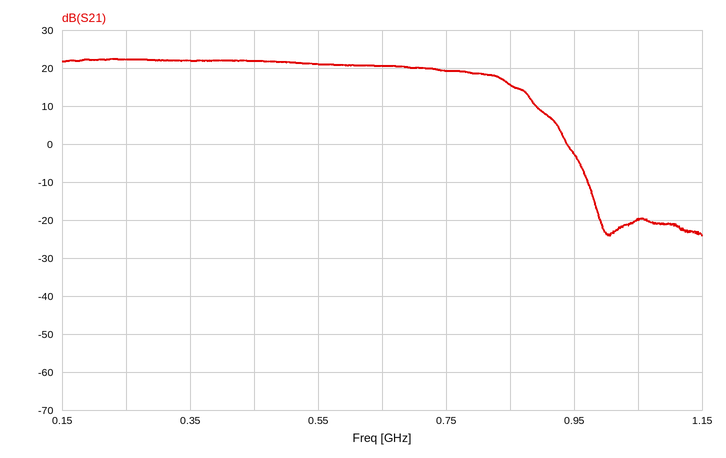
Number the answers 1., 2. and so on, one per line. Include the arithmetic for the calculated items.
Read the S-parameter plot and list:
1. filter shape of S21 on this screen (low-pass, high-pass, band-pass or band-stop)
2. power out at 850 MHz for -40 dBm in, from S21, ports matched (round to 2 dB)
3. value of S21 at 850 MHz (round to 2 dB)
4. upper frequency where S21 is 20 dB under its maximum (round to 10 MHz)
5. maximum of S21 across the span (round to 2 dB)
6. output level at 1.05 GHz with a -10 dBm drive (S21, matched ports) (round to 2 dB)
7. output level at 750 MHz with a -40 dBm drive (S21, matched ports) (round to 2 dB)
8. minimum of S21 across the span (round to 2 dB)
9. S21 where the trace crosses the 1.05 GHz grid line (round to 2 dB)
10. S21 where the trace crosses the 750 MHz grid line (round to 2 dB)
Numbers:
1. low-pass
2. -40 dBm + (16 dB) = -24 dBm
3. 16 dB
4. 930 MHz
5. 22 dB
6. -10 dBm + (-20 dB) = -30 dBm
7. -40 dBm + (20 dB) = -20 dBm
8. -24 dB
9. -20 dB
10. 20 dB
